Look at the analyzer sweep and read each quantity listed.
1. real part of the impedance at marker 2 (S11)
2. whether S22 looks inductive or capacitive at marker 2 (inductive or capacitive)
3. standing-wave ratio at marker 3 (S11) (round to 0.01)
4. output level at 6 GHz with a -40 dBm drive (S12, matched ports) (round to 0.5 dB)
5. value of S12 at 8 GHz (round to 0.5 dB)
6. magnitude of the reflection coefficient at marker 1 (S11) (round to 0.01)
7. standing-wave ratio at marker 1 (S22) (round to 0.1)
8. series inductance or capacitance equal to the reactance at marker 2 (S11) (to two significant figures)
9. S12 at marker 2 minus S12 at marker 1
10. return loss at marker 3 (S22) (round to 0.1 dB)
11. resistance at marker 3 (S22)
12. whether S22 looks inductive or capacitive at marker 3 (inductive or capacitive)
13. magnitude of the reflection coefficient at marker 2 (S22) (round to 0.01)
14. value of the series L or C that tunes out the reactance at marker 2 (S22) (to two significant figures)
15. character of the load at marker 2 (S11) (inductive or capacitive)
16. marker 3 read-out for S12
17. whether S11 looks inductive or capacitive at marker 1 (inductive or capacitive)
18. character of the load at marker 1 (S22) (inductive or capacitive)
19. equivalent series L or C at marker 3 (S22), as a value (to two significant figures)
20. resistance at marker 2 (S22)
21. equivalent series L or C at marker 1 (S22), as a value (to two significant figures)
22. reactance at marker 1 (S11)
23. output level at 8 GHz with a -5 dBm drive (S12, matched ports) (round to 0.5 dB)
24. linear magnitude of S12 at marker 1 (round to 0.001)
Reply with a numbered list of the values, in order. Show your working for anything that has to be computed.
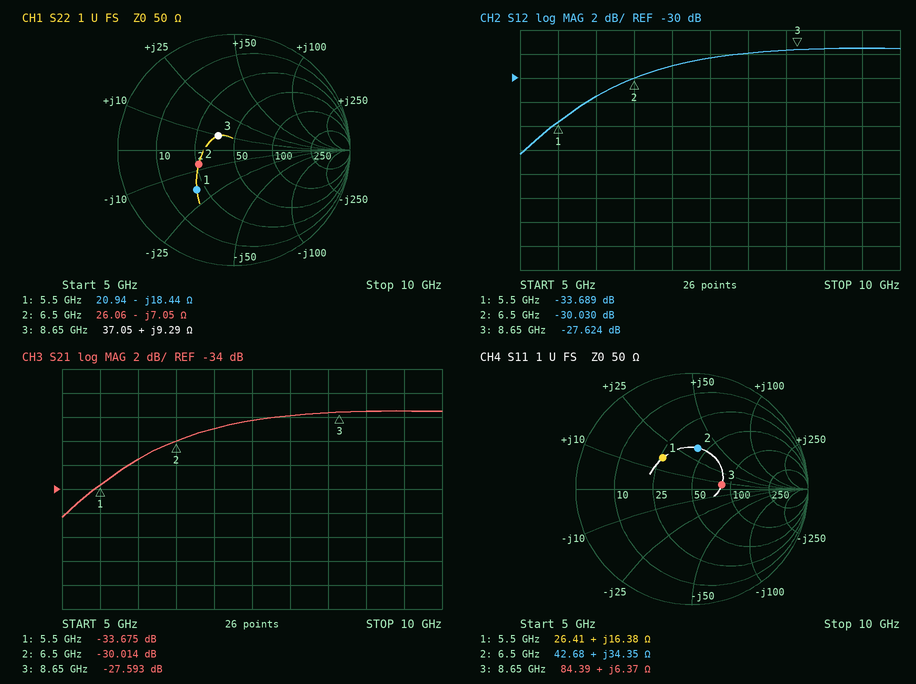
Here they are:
1. 42.68 Ω
2. capacitive
3. 1.70
4. -40 dBm + (-31.5 dB) = -71.5 dBm
5. -28.0 dB
6. 0.37
7. 2.8
8. L = 34.35 Ω/(2π × 6.5 GHz) ≈ 841 pH, so 840 pH to two significant figures
9. -30.03 − (-33.689) = 3.659 dB
10. 14.8 dB
11. 37.05 Ω
12. inductive
13. 0.33
14. L = 7.05 Ω/(2π × 6.5 GHz) ≈ 173 pH, so 170 pH to two significant figures
15. inductive
16. -27.624 dB
17. inductive
18. capacitive
19. L = 9.29 Ω/(2π × 8.65 GHz) ≈ 171 pH, so 170 pH to two significant figures
20. 26.06 Ω
21. C = 1/(2π × 5.5 GHz × 18.44 Ω) ≈ 1.6 pF
22. +16.38 Ω
23. -5 dBm + (-28.0 dB) = -33.0 dBm
24. 10^(-33.689/20) ≈ 0.021
